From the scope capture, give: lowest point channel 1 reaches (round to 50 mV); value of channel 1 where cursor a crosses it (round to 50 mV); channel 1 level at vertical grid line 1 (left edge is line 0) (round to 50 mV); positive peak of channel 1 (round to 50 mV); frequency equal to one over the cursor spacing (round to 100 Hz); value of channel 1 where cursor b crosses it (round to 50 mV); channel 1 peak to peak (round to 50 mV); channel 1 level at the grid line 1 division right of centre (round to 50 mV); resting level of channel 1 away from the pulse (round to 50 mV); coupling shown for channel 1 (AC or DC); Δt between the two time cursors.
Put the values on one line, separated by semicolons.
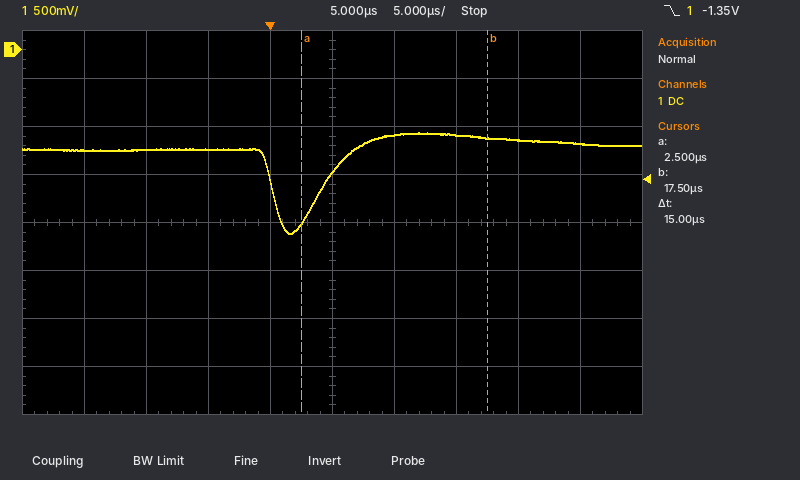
-1.90 V; -1.80 V; -1.05 V; -850 mV; 66.7 kHz; -900 mV; 1.05 V; -900 mV; -1.05 V; DC; 15 µs
